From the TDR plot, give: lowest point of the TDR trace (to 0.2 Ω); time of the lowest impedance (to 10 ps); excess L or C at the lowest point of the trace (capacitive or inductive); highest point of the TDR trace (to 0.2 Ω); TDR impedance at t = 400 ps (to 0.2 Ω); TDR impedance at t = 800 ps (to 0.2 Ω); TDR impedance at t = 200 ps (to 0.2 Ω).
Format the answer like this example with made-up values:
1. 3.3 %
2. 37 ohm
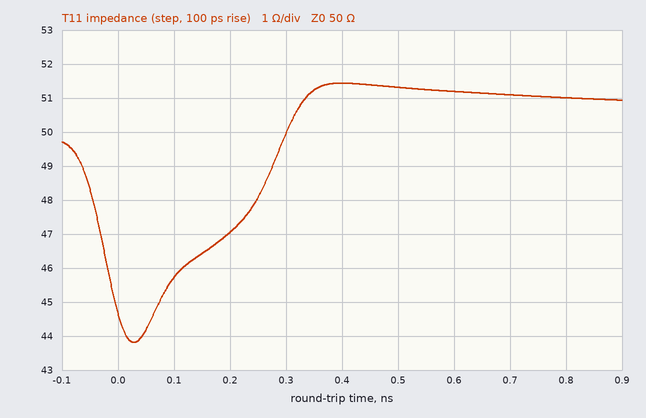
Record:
1. 43.8 Ω
2. 30 ps
3. capacitive
4. 51.4 Ω
5. 51.4 Ω
6. 51.0 Ω
7. 47.0 Ω
